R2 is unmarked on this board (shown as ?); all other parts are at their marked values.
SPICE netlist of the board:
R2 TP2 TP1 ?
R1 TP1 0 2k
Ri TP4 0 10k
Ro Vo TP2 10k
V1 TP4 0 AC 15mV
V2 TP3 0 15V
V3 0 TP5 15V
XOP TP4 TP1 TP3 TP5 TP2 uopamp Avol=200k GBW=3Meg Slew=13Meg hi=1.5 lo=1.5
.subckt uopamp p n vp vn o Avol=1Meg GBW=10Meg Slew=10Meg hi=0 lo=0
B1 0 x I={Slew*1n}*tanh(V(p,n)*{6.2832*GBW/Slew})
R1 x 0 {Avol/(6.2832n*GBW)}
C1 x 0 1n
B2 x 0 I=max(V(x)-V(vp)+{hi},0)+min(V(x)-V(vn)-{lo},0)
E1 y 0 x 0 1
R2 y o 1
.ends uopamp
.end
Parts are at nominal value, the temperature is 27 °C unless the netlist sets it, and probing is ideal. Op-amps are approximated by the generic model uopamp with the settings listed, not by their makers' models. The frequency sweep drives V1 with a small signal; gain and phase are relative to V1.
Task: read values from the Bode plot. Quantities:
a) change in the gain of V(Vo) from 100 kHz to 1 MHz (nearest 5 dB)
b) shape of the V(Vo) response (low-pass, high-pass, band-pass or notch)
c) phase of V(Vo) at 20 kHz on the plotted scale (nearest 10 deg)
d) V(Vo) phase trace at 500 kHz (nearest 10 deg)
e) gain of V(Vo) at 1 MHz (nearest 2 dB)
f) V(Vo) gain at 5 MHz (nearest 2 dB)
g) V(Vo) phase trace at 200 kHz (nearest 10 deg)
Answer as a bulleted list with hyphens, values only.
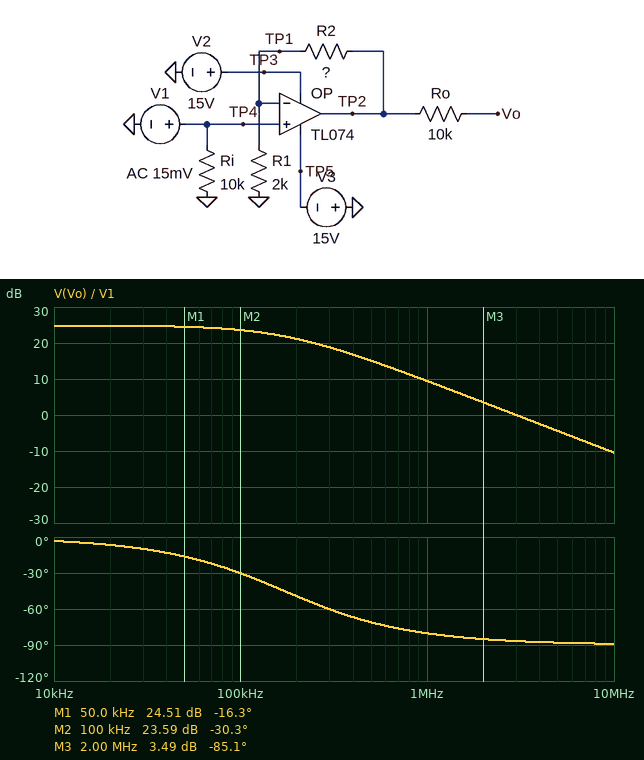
- -15 dB
- low-pass
- -10 deg
- -70 deg
- 10 dB
- -4 dB
- -50 deg
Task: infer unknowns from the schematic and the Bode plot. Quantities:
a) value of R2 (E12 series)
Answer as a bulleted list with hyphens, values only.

- 33 kΩ
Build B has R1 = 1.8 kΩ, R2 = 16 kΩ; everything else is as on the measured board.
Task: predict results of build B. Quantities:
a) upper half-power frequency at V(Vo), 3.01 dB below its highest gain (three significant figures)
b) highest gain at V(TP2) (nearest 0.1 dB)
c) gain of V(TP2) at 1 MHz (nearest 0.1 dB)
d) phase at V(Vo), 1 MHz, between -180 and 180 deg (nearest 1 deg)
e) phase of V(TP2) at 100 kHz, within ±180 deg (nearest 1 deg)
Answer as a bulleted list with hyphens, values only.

- 303 kHz
- 19.9 dB
- 9.2 dB
- -73 deg
- -18 deg
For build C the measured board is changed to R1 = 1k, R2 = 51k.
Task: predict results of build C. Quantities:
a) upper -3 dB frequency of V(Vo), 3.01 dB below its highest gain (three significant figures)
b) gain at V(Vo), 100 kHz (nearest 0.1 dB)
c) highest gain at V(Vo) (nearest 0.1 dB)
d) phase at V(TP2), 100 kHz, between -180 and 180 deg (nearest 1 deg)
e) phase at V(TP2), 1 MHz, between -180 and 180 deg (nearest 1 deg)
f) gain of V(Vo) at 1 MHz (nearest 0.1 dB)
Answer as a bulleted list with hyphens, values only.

- 57.7 kHz
- 28.3 dB
- 34.3 dB
- -60 deg
- -87 deg
- 9.5 dB
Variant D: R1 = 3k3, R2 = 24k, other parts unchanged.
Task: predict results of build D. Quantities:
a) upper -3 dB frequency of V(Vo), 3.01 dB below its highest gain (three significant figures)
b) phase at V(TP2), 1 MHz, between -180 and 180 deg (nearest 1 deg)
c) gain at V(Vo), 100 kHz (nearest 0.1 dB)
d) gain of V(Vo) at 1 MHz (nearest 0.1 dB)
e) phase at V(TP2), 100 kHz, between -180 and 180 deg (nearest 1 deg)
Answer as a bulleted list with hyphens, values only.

- 363 kHz
- -70 deg
- 18.0 dB
- 9.0 dB
- -15 deg
